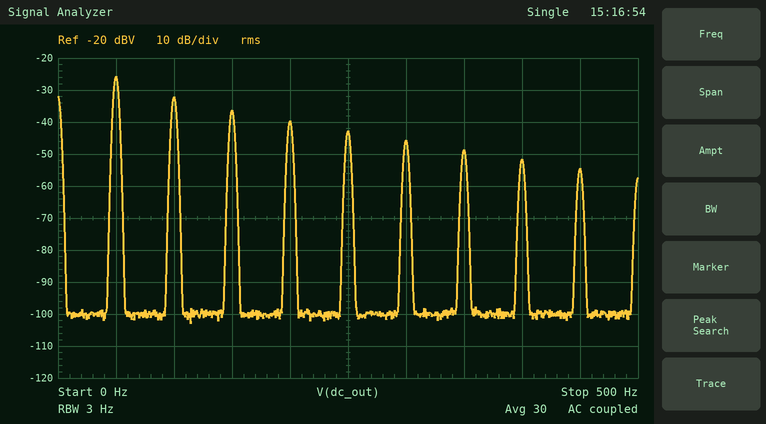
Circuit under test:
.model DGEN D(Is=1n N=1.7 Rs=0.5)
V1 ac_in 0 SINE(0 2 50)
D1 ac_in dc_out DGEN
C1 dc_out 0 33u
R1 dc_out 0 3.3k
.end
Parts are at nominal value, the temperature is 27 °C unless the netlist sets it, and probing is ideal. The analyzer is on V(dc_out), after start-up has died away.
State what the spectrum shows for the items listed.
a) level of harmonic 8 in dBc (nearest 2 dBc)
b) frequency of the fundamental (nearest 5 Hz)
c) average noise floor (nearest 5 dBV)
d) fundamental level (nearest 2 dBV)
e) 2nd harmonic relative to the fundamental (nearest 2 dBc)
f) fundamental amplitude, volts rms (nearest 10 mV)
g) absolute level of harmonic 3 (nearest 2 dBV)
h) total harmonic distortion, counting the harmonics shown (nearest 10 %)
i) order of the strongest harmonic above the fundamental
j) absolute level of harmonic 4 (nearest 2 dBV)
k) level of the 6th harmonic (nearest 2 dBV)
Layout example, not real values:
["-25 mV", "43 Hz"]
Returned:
["-26 dBc", "50 Hz", "-100 dBV", "-26 dBV", "-6 dBc", "50 mV", "-36 dBV", "60 %", "2", "-40 dBV", "-46 dBV"]
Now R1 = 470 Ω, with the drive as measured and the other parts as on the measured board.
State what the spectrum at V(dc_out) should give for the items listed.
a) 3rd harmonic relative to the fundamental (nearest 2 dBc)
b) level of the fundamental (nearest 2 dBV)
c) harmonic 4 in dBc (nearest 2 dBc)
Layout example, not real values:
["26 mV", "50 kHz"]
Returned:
["-12 dBc", "-12 dBV", "-18 dBc"]
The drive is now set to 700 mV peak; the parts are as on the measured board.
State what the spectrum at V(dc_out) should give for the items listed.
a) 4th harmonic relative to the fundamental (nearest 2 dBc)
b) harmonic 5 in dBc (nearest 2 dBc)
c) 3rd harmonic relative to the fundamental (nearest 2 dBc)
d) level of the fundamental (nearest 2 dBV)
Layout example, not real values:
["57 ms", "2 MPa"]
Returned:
["-16 dBc", "-20 dBc", "-12 dBc", "-46 dBV"]
